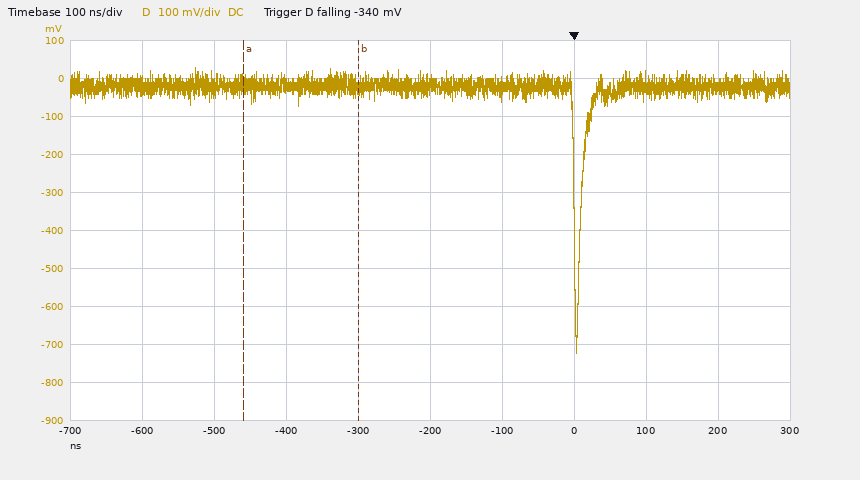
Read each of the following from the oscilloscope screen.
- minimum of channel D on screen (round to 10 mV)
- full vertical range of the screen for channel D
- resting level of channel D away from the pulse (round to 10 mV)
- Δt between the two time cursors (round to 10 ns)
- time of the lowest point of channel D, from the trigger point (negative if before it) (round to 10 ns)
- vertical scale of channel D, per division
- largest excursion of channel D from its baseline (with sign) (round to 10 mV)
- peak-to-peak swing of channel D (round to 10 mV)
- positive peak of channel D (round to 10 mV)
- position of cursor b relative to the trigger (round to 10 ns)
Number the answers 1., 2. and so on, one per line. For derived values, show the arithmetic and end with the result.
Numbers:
1. -720 mV
2. 1 V
3. -20 mV
4. 160 ns
5. 0 ns
6. 100 mV
7. -720 mV − (-20 mV) = -700 mV
8. 30 mV − (-720 mV) = 750 mV
9. 30 mV
10. -300 ns
